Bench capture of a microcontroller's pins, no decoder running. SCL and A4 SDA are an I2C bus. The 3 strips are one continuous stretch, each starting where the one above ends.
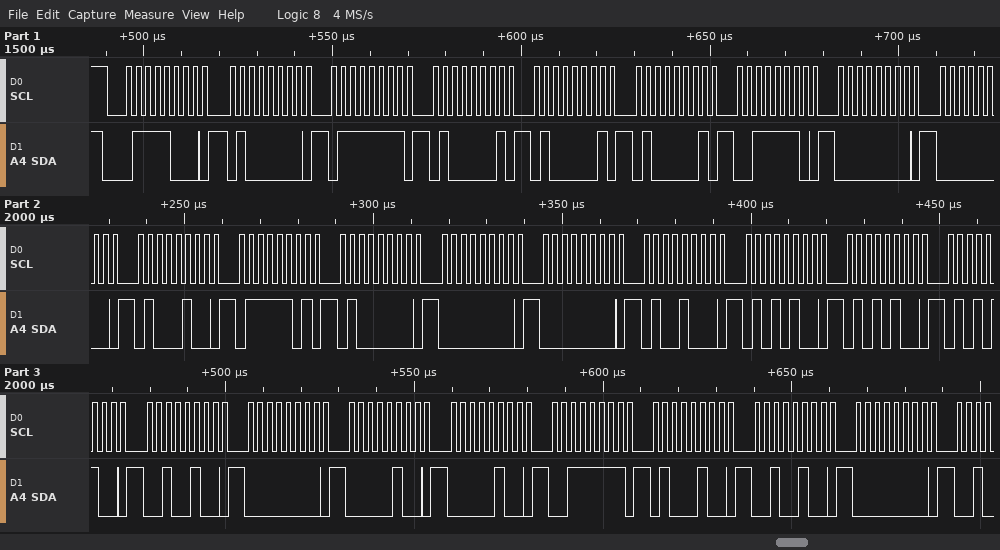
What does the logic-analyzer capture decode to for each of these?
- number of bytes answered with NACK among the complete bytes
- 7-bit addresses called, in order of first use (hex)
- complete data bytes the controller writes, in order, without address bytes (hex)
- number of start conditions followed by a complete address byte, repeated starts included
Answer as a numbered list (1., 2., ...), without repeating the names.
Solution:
1. 0
2. 0x3C
3. 40 7F 41 41 41 3E 00 00 44 7D 40 00 00 48 54 54 54 24 00 04 04 3F 44 24 00
4. 1
